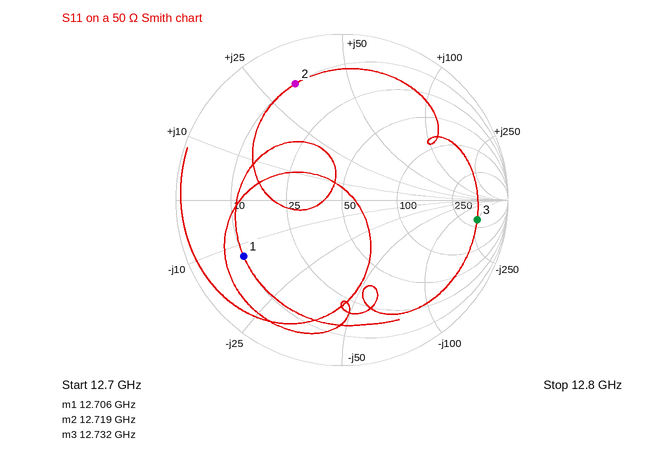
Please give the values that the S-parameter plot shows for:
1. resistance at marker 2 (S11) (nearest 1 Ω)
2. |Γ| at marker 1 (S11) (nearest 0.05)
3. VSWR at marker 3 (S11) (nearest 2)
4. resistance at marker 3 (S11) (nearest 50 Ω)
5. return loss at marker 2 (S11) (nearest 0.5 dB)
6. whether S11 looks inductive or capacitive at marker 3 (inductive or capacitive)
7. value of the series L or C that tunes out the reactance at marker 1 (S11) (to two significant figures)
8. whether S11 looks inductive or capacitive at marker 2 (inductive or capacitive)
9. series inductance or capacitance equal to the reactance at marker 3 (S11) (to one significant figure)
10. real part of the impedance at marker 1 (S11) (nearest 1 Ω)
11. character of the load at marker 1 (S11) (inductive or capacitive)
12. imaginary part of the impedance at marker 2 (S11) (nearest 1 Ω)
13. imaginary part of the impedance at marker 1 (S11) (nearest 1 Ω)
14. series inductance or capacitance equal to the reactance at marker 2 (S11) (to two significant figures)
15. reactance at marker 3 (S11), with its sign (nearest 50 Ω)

10 Ω
0.70
10
350 Ω
2.5 dB
capacitive
160 pH
inductive
50 fF
10 Ω
capacitive
+33 Ω
-13 Ω
410 pH
-250 Ω
